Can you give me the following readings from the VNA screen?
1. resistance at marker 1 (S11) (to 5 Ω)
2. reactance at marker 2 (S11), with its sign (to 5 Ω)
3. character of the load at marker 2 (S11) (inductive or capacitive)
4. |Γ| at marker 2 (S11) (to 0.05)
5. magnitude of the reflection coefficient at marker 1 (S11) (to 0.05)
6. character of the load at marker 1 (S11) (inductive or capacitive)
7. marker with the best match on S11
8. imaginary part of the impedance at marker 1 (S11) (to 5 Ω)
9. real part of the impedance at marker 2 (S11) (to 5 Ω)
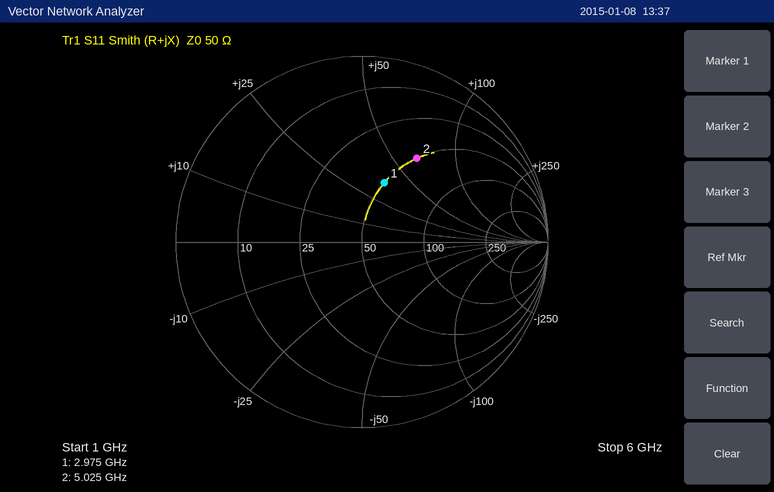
50 Ω
+65 Ω
inductive
0.55
0.35
inductive
marker 1
+35 Ω
50 Ω
